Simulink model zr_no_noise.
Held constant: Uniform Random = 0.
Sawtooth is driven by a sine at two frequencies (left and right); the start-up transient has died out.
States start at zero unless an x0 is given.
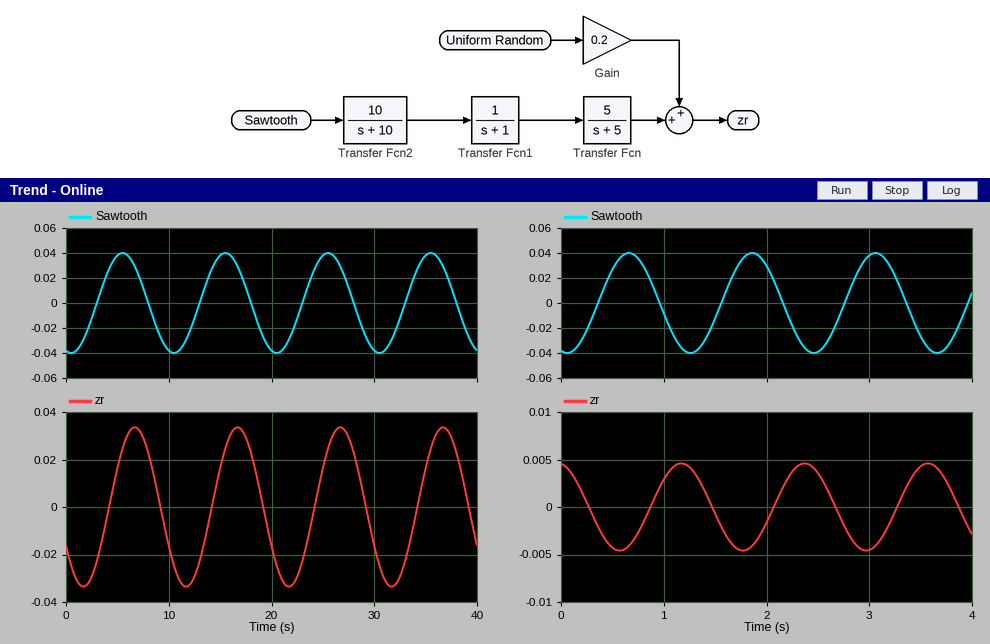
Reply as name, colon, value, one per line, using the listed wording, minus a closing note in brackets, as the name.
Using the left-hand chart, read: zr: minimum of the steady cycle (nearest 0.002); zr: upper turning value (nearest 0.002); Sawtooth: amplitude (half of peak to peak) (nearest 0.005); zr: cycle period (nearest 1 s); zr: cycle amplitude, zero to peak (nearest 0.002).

zr: minimum of the steady cycle: -0.034
zr: upper turning value: 0.034
Sawtooth: amplitude (half of peak to peak): 0.040
zr: cycle period: 10 s
zr: cycle amplitude, zero to peak: 0.034
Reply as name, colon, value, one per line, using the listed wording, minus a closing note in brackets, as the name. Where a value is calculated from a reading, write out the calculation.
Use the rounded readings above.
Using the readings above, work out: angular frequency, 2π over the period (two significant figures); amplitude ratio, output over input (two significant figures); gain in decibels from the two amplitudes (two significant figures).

angular frequency, 2π over the period: 2π / 10 = 0.63 rad/s
amplitude ratio, output over input: 0.034 / 0.04 = 0.85
gain in decibels from the two amplitudes: 20 log10(0.034 / 0.04) = -1.4 dB
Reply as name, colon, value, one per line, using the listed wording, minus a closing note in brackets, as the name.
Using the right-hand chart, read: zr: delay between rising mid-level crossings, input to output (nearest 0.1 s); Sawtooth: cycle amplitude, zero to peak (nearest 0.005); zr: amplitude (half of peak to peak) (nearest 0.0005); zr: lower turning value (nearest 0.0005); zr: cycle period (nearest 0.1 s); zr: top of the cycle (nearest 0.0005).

zr: delay between rising mid-level crossings, input to output: 0.5 s
Sawtooth: cycle amplitude, zero to peak: 0.040
zr: amplitude (half of peak to peak): 0.0045
zr: lower turning value: -0.0045
zr: cycle period: 1.2 s
zr: top of the cycle: 0.0045
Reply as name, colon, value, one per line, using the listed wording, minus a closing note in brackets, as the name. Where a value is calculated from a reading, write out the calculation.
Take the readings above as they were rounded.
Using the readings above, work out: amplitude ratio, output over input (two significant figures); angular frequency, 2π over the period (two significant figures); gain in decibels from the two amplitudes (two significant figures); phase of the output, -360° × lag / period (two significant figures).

amplitude ratio, output over input: 0.0045 / 0.04 = 0.11
angular frequency, 2π over the period: 2π / 1.2 = 5.2 rad/s
gain in decibels from the two amplitudes: 20 log10(0.0045 / 0.04) = -19 dB
phase of the output, -360° × lag / period: -360 × 0.5 / 1.2 = -150°
